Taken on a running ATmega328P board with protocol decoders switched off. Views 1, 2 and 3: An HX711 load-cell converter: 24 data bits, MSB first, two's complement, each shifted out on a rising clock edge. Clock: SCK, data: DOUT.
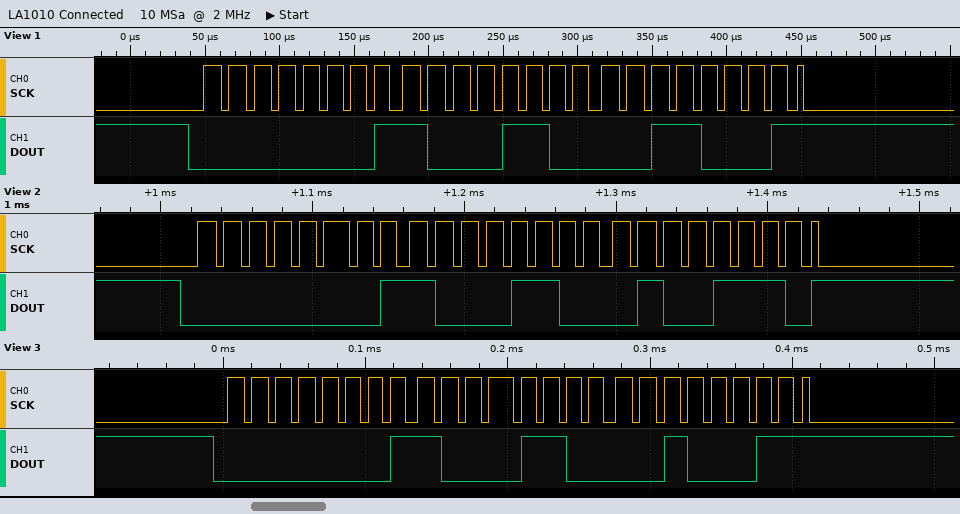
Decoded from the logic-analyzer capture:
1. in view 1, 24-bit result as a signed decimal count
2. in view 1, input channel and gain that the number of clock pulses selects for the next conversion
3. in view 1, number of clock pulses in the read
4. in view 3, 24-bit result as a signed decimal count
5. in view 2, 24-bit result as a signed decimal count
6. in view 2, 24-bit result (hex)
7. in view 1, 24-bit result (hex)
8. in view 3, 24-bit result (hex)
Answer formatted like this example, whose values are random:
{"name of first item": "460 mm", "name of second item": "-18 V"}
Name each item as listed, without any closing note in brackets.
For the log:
{"in view 1, 24-bit result as a signed decimal count": "101425", "in view 1, input channel and gain that the number of clock pulses selects for the next conversion": "channel A, gain 128", "in view 1, number of clock pulses in the read": "25", "in view 3, 24-bit result as a signed decimal count": "101411", "in view 2, 24-bit result as a signed decimal count": "101454", "in view 2, 24-bit result": "0x018C4E", "in view 1, 24-bit result": "0x018C31", "in view 3, 24-bit result": "0x018C23"}
